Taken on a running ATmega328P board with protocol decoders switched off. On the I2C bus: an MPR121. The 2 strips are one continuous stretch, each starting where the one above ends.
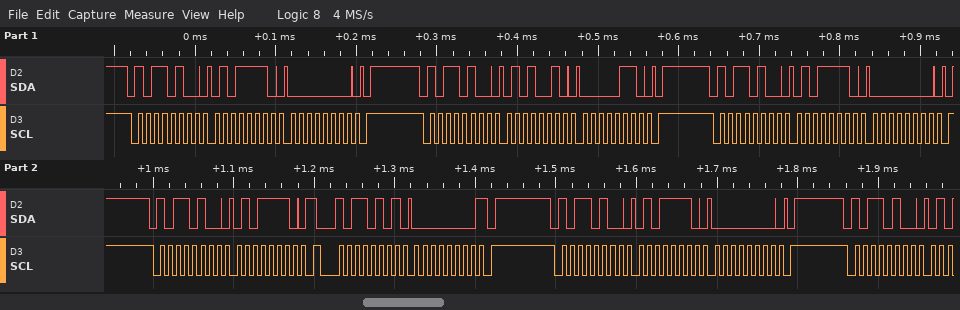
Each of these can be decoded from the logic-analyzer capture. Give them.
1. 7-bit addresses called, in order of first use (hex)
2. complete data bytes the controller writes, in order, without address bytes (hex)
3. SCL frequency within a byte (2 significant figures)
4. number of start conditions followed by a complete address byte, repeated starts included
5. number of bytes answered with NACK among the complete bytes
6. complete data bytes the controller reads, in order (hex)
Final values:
0x5A
5E 00 52 06 5E 00 5E 5E 00
100 kHz
7
1
00
